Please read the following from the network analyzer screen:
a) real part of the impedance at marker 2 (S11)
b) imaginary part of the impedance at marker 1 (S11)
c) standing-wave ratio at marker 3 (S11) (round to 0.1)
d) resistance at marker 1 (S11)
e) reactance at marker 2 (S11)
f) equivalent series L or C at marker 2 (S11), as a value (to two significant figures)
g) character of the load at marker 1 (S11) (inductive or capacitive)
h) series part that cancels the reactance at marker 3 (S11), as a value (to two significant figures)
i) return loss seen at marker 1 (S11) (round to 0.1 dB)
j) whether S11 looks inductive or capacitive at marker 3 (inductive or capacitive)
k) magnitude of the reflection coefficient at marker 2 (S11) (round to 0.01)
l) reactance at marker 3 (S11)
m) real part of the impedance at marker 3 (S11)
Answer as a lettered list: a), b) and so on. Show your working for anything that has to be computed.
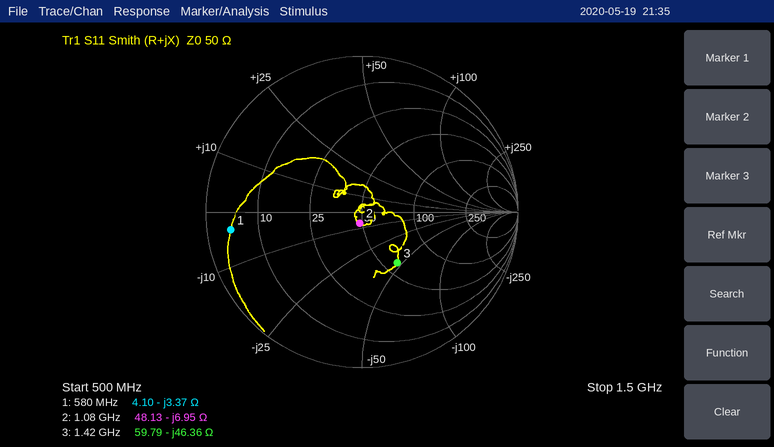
a) 48.13 Ω
b) -3.37 Ω
c) 2.3
d) 4.10 Ω
e) -6.95 Ω
f) C = 1/(2π × 1.08 GHz × 6.95 Ω) ≈ 21 pF
g) capacitive
h) L = 46.36 Ω/(2π × 1.42 GHz) ≈ 5.2 nH
i) 1.4 dB
j) capacitive
k) 0.07
l) -46.36 Ω
m) 59.79 Ω
